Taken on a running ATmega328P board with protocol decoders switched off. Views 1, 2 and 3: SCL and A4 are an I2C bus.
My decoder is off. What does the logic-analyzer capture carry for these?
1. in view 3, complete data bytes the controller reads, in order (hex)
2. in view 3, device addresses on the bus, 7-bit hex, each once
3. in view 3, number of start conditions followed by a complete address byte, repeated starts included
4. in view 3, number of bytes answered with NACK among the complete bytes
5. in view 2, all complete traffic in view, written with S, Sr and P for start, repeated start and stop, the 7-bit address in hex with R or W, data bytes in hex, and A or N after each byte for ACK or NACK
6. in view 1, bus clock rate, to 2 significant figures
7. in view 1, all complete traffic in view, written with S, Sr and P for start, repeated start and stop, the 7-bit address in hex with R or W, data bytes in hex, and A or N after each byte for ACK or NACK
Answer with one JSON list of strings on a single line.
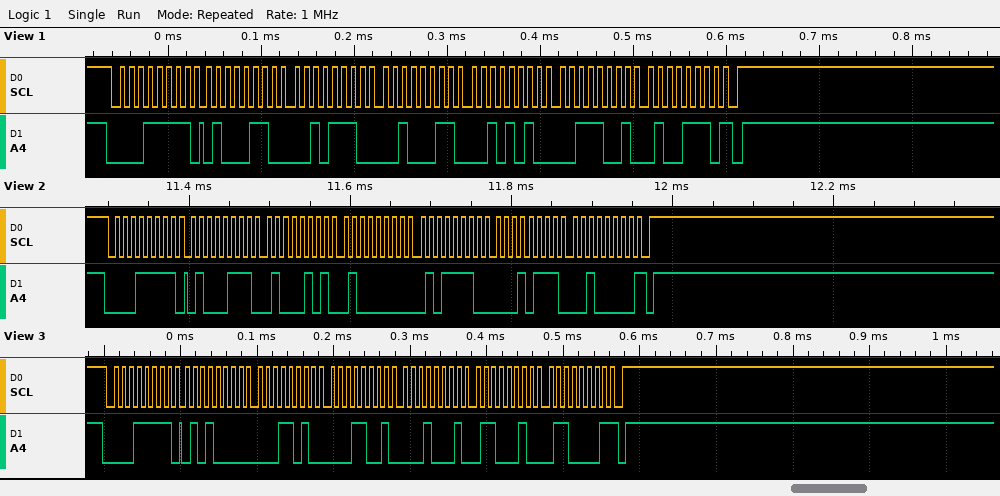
["50 1A 19 11 62 61", "0x0F", "1", "1", "S 0FR A 47 A 45 A 40 A 5E A 17 A 20 N P", "100 kHz", "S 0FR A 46 A 2E A 23 A 2A A 39 A 4E N P"]
